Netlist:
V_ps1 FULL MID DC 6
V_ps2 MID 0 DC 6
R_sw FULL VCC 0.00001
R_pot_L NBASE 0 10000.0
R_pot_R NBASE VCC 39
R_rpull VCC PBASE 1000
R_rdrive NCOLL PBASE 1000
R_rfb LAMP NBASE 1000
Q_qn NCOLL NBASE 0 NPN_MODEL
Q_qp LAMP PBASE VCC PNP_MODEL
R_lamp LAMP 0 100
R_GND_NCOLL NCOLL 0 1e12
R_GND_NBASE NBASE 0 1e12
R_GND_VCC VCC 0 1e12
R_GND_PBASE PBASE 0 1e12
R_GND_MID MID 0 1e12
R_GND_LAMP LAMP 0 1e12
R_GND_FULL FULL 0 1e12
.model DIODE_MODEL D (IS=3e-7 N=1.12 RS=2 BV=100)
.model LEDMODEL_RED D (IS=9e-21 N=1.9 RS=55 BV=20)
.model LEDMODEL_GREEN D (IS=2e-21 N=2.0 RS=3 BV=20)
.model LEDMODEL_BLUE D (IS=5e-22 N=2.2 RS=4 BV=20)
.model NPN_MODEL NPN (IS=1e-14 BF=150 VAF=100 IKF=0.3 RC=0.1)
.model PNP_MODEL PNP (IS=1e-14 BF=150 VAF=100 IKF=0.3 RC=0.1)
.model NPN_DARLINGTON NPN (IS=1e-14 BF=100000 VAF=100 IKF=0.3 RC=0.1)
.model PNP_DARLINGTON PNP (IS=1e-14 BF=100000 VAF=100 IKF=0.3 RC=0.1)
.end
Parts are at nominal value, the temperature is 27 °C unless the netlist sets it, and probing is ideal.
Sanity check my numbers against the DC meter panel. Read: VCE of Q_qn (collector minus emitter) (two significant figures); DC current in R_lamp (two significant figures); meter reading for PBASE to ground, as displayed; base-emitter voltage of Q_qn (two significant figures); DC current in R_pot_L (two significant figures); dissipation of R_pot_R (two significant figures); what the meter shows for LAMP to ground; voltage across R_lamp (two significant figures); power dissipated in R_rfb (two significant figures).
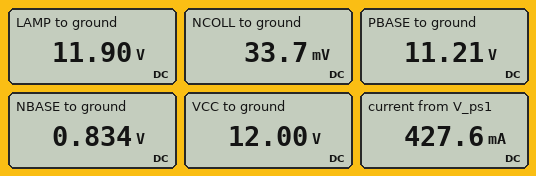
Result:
34 mV
120 mA
11.21 V
830 mV
83 µA
3.2 W
11.90 V
12 V
120 mW
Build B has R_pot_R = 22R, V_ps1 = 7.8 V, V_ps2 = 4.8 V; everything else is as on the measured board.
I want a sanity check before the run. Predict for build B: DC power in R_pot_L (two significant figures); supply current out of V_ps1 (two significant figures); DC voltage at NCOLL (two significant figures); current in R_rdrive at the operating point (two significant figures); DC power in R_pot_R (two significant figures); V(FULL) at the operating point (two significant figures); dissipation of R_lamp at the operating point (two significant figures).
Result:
73 µW
680 mA
40 mV
12 mA
6.3 W
13 V
1.6 W
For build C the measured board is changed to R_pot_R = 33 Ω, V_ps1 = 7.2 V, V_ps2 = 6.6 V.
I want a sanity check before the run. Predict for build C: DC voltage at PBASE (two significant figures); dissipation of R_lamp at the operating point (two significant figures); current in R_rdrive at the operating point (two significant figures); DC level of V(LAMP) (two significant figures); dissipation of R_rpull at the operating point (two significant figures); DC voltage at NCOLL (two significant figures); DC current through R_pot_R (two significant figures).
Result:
13 V
1.9 W
13 mA
14 V
640 µW
37 mV
390 mA
